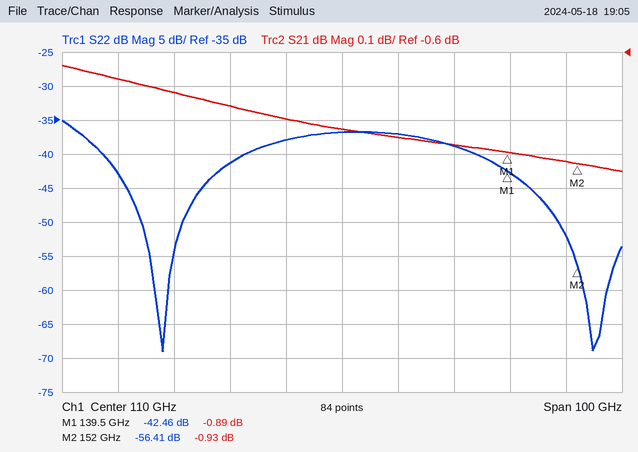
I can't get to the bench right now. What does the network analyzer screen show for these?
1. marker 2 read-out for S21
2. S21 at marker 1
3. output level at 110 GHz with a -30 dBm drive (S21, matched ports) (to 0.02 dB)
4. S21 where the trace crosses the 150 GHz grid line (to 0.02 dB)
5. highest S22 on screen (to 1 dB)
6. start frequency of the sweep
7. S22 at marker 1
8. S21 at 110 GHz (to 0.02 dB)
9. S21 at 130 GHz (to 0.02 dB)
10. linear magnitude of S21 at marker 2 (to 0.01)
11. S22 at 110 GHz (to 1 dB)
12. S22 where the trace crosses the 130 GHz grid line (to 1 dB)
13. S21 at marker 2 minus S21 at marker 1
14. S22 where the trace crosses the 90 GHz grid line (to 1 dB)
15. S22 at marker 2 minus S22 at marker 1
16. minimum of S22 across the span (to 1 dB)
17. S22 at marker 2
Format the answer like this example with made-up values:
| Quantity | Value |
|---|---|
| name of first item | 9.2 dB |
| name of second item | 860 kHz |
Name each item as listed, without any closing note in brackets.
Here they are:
| Quantity | Value |
|---|---|
| marker 2 read-out for S21 | -0.93 dB |
| S21 at marker 1 | -0.89 dB |
| output level at 110 GHz with a -30 dBm drive (S21, matched ports) | -30.82 dBm |
| S21 where the trace crosses the 150 GHz grid line | -0.92 dB |
| highest S22 on screen | -35 dB |
| start frequency of the sweep | 60 GHz |
| S22 at marker 1 | -42.46 dB |
| S21 at 110 GHz | -0.82 dB |
| S21 at 130 GHz | -0.88 dB |
| linear magnitude of S21 at marker 2 | 0.90 |
| S22 at 110 GHz | -37 dB |
| S22 where the trace crosses the 130 GHz grid line | -39 dB |
| S21 at marker 2 minus S21 at marker 1 | -0.04 dB |
| S22 where the trace crosses the 90 GHz grid line | -41 dB |
| S22 at marker 2 minus S22 at marker 1 | -13.95 dB |
| minimum of S22 across the span | -69 dB |
| S22 at marker 2 | -56.41 dB |
